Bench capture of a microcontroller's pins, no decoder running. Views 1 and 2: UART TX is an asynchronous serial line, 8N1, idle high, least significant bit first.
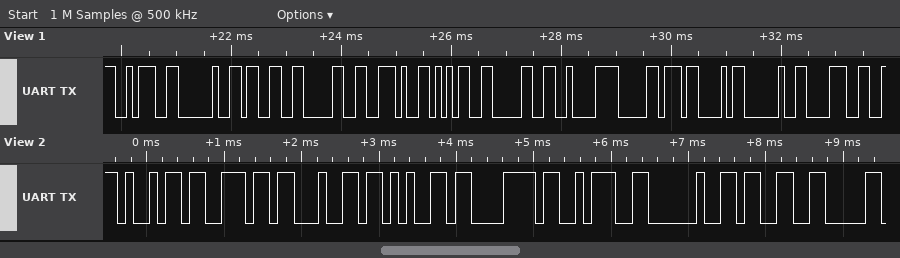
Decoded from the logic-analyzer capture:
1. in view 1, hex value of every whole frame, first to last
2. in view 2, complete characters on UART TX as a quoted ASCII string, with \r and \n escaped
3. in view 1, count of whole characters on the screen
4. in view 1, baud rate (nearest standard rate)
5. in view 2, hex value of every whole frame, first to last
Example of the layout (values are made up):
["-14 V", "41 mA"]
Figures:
["3A 20 33 30 2E 35 30 C2 B0 43 20 38", "\"index: 3\"", "12", "9600 baud", "69 6E 64 65 78 3A 20 33"]
